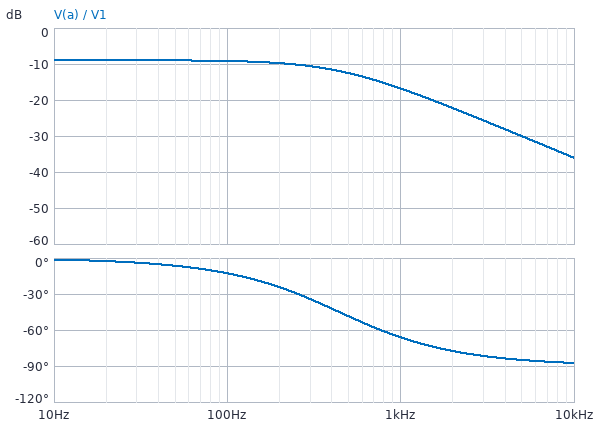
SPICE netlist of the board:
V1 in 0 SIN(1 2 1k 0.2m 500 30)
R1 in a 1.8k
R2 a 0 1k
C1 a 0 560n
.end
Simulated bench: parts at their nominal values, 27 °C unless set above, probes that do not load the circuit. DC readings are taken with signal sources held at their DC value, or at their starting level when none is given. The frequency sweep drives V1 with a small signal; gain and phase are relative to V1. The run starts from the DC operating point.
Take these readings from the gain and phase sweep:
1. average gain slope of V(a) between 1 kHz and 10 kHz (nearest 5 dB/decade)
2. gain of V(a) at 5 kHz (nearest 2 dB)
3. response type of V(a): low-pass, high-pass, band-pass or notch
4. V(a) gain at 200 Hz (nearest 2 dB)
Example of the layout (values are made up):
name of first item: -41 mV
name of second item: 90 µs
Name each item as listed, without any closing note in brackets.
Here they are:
average gain slope of V(a) between 1 kHz and 10 kHz: -20 dB/decade
gain of V(a) at 5 kHz: -30 dB
response type of V(a): low-pass, high-pass, band-pass or notch: low-pass
V(a) gain at 200 Hz: -10 dB
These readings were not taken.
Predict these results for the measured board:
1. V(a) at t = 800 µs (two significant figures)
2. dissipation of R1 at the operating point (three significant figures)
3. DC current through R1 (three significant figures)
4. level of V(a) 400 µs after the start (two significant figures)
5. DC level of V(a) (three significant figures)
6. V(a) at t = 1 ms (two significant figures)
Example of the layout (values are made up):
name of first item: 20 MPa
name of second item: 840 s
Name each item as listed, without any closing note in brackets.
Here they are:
V(a) at t = 800 µs: 480 mV
dissipation of R1 at the operating point: 918 µW
DC current through R1: 714 µA
level of V(a) 400 µs after the start: 810 mV
DC level of V(a): 714 mV
V(a) at t = 1 ms: 230 mV
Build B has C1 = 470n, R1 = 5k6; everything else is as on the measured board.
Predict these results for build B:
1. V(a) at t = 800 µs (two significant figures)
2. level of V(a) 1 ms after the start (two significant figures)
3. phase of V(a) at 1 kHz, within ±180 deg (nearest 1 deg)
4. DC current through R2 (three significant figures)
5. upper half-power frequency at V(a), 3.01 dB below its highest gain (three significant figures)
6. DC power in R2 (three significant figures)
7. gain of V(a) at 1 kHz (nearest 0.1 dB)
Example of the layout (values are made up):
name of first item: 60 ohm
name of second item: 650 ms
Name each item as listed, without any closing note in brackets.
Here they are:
V(a) at t = 800 µs: 210 mV
level of V(a) 1 ms after the start: 110 mV
phase of V(a) at 1 kHz, within ±180 deg: -68 deg
DC current through R2: 303 µA
upper half-power frequency at V(a), 3.01 dB below its highest gain: 399 Hz
DC power in R2: 91.8 µW
gain of V(a) at 1 kHz: -25.0 dB
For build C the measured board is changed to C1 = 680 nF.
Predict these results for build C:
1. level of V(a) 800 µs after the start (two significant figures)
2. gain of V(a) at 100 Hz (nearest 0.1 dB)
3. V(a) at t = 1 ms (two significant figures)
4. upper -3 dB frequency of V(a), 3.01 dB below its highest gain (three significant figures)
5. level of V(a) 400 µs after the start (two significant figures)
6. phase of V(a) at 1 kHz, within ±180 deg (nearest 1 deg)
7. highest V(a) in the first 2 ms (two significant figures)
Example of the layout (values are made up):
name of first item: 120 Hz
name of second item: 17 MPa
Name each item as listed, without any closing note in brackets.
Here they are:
level of V(a) 800 µs after the start: 520 mV
gain of V(a) at 100 Hz: -9.3 dB
V(a) at t = 1 ms: 290 mV
upper -3 dB frequency of V(a), 3.01 dB below its highest gain: 364 Hz
level of V(a) 400 µs after the start: 800 mV
phase of V(a) at 1 kHz, within ±180 deg: -70 deg
highest V(a) in the first 2 ms: 820 mV
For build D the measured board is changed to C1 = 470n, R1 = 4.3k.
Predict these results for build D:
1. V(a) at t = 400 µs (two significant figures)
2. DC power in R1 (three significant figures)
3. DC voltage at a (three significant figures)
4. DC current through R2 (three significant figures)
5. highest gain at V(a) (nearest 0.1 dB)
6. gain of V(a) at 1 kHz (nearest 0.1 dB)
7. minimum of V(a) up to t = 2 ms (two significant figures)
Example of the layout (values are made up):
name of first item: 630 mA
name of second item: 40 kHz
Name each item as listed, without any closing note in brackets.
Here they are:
V(a) at t = 400 µs: 430 mV
DC power in R1: 612 µW
DC voltage at a: 377 mV
DC current through R2: 377 µA
highest gain at V(a): -14.5 dB
gain of V(a) at 1 kHz: -22.8 dB
minimum of V(a) up to t = 2 ms: 120 mV
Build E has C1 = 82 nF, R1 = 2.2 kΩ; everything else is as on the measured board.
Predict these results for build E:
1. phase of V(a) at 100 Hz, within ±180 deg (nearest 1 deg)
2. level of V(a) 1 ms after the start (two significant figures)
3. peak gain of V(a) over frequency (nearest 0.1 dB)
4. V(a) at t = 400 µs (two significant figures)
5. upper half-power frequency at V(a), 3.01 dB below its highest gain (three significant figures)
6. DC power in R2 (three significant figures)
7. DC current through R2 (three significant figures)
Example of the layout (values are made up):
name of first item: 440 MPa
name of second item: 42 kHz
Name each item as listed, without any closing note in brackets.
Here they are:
phase of V(a) at 100 Hz, within ±180 deg: -2 deg
level of V(a) 1 ms after the start: -45 mV
peak gain of V(a) over frequency: -10.1 dB
V(a) at t = 400 µs: 860 mV
upper half-power frequency at V(a), 3.01 dB below its highest gain: 2.82 kHz
DC power in R2: 391 µW
DC current through R2: 625 µA
